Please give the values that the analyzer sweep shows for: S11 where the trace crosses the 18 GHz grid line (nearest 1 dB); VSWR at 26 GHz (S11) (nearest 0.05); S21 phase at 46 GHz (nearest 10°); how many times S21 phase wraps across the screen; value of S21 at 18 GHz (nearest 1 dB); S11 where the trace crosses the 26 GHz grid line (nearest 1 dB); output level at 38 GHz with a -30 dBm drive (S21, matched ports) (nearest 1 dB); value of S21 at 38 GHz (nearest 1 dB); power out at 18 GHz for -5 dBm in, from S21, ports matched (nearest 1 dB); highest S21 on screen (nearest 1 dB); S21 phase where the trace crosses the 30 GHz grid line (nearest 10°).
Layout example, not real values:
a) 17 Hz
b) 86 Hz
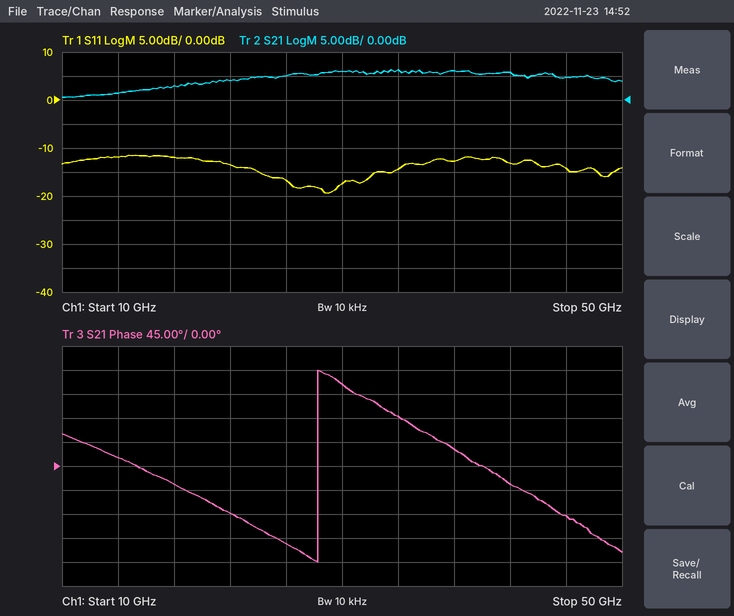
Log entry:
a) -12 dB
b) 1.35
c) -90°
d) 1
e) 3 dB
f) -17 dB
g) -24 dBm
h) 6 dB
i) -2 dBm
j) 6 dB
k) 150°
